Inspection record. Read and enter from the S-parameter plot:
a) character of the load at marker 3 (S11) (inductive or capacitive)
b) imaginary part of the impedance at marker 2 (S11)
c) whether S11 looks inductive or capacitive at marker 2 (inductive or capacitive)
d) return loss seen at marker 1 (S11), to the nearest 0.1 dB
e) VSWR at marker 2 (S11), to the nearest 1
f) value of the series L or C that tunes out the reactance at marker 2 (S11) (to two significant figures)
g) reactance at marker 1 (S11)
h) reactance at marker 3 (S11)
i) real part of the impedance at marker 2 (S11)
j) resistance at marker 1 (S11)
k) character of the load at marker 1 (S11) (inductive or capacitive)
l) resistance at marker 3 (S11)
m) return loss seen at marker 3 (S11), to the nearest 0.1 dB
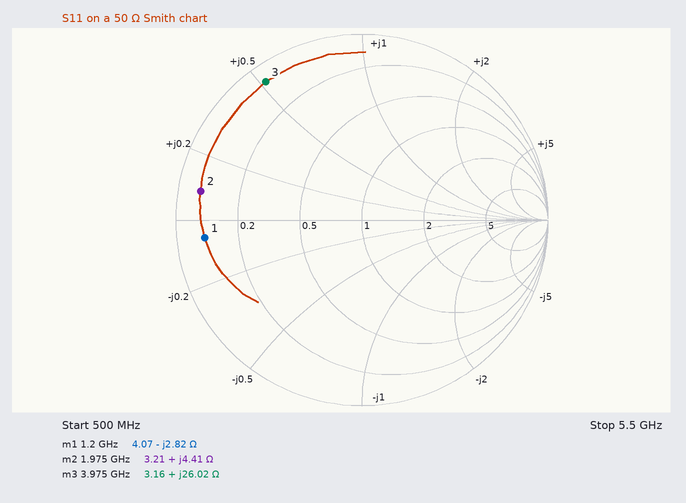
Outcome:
inductive
+4.41 Ω
inductive
1.4 dB
16
18 pF
-2.82 Ω
+26.02 Ω
3.21 Ω
4.07 Ω
capacitive
3.16 Ω
0.9 dB
